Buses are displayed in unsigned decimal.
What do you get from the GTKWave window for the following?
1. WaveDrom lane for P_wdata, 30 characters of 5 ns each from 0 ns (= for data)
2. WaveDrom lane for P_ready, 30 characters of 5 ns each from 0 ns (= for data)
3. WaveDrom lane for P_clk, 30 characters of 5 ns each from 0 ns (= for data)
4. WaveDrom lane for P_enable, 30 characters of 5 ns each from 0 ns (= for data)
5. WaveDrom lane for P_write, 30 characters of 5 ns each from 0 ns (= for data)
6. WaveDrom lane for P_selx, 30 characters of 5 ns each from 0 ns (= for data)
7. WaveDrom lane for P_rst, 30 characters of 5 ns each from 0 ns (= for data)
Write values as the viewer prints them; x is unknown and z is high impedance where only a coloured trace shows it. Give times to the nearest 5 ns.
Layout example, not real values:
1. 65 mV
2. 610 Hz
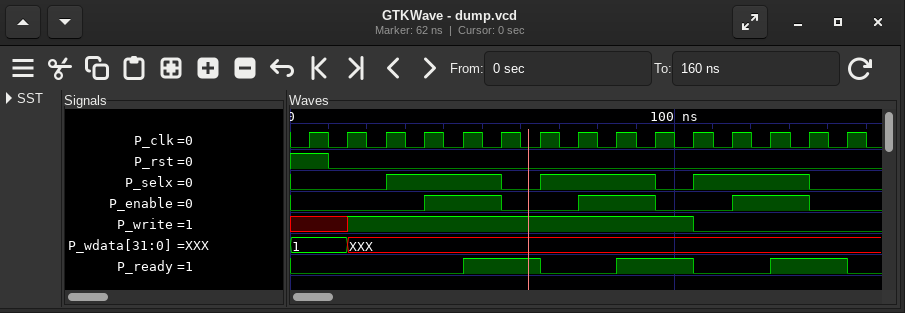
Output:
1. {name: 'P_wdata', wave: '=..x..........................', data: '1'}
2. {name: 'P_ready', wave: '0........1...0...1...0...1...0'}
3. {name: 'P_clk', wave: '010101010101010101010101010101'}
4. {name: 'P_enable', wave: '0......1...0...1...0...1...0..'}
5. {name: 'P_write', wave: 'x..1.................0........'}
6. {name: 'P_selx', wave: '0....1.....0.1.....0.1.....0..'}
7. {name: 'P_rst', wave: '1.0...........................'}
